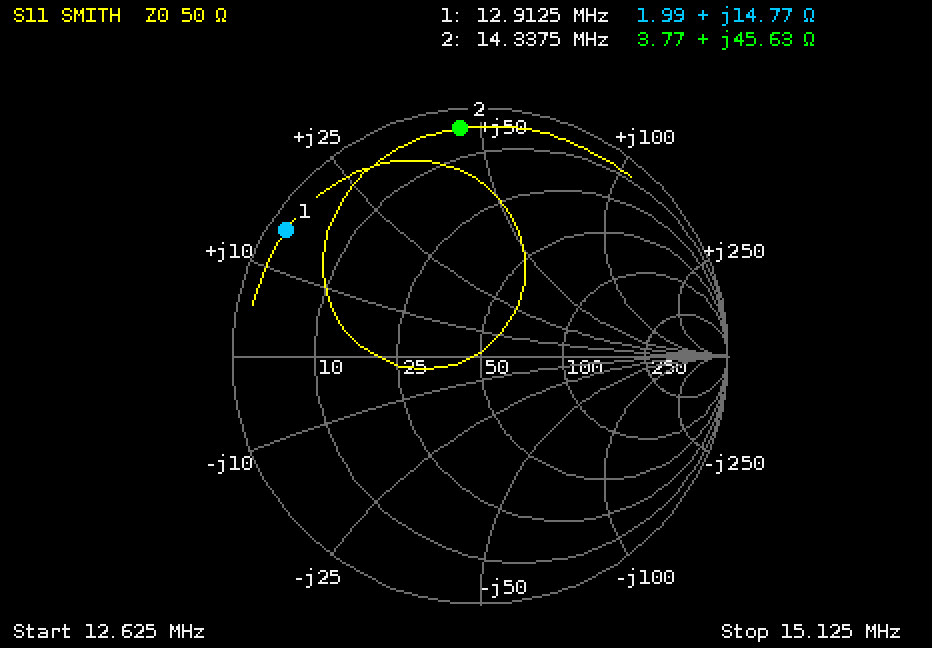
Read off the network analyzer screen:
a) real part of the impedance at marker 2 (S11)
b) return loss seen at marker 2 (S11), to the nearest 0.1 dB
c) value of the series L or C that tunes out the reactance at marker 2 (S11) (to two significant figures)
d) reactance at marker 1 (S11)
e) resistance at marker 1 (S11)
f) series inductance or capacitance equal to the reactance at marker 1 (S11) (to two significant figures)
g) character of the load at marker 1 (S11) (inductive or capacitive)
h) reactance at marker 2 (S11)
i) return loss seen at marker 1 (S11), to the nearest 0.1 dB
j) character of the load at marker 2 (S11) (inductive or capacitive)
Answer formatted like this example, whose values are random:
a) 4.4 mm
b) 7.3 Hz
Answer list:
a) 3.77 Ω
b) 0.7 dB
c) 240 pF
d) +14.77 Ω
e) 1.99 Ω
f) 180 nH
g) inductive
h) +45.63 Ω
i) 0.6 dB
j) inductive
